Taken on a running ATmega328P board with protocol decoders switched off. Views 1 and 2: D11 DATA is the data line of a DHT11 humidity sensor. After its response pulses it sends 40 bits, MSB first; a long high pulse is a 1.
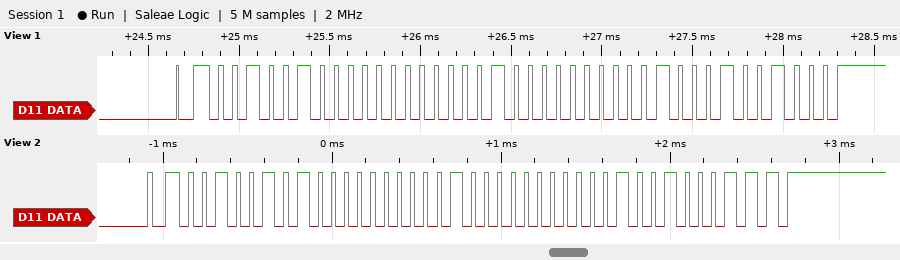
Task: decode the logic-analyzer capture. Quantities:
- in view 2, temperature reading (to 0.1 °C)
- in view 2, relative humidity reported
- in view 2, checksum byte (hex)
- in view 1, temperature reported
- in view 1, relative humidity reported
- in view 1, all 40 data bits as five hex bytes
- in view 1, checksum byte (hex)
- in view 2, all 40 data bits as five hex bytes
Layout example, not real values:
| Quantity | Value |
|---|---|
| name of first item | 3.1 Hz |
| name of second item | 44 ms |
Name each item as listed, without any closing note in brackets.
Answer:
| Quantity | Value |
|---|---|
| in view 2, temperature reading | 32.2 °C |
| in view 2, relative humidity reported | 37 % |
| in view 2, checksum byte | 0x47 |
| in view 1, temperature reported | 32.4 °C |
| in view 1, relative humidity reported | 36 % |
| in view 1, all 40 data bits as five hex bytes | 24 00 20 04 48 |
| in view 1, checksum byte | 0x48 |
| in view 2, all 40 data bits as five hex bytes | 25 00 20 02 47 |
